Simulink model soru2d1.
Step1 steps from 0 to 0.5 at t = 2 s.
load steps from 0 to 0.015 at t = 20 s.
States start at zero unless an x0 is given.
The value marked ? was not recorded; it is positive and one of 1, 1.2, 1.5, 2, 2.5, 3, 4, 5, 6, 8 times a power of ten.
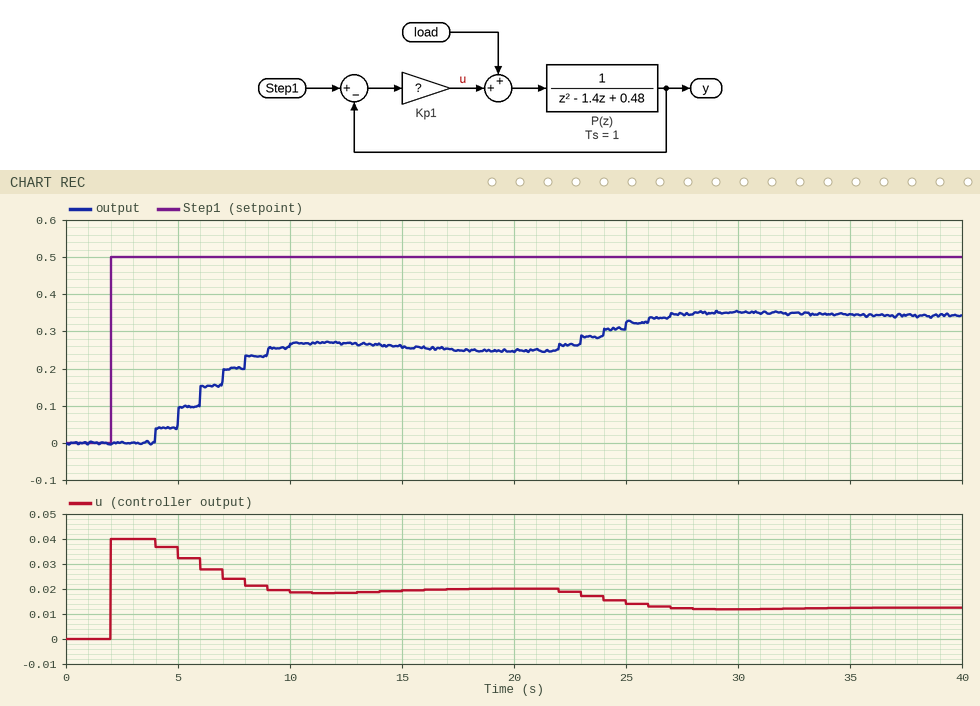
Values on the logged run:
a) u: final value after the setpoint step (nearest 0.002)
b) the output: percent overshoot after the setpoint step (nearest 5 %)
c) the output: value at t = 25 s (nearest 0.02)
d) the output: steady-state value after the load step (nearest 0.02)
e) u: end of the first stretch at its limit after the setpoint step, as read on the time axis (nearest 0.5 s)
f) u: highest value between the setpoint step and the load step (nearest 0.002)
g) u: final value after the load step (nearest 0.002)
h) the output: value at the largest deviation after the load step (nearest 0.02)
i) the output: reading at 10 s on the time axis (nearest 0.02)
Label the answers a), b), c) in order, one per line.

a) 0.020
b) 10 %
c) 0.32
d) 0.34
e) 4.0 s
f) 0.040
g) 0.012
h) 0.36
i) 0.26
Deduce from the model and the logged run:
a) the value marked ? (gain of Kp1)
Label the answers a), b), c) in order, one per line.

a) 0.08
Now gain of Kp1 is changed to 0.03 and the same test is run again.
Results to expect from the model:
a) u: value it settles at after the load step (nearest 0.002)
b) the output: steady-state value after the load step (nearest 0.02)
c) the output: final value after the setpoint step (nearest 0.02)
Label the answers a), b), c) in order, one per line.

a) 0.006
b) 0.28
c) 0.14
